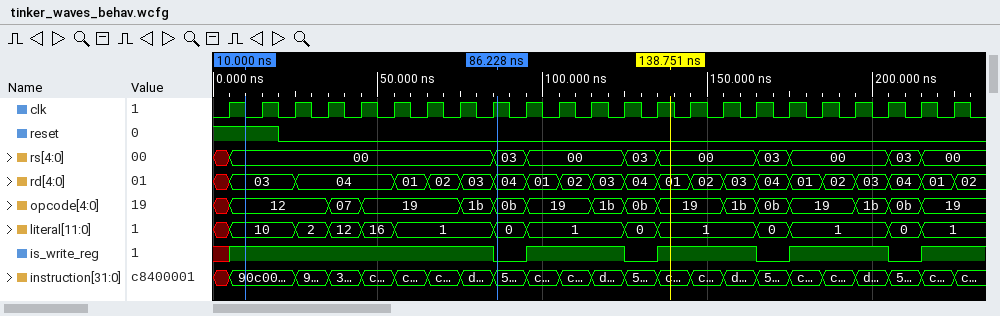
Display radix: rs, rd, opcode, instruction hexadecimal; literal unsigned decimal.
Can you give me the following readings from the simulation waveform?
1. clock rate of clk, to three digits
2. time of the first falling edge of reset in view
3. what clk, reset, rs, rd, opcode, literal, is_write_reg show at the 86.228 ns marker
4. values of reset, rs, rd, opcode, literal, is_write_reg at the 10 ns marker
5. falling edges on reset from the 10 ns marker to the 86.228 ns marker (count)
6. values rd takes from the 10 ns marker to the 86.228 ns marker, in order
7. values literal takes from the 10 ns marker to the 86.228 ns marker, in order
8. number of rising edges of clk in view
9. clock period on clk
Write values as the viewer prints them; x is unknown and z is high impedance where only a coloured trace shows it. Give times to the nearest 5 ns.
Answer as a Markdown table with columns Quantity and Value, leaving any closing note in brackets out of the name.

| Quantity | Value |
|---|---|
| clock rate of clk, to three digits | 100 MHz |
| time of the first falling edge of reset in view | 20 ns |
| what clk, reset, rs, rd, opcode, literal, is_write_reg show at the 86.228 ns marker | clk=1, reset=0, rs=03, rd=04, opcode=0b, literal=0, is_write_reg=0 |
| values of reset, rs, rd, opcode, literal, is_write_reg at the 10 ns marker | reset=1, rs=00, rd=03, opcode=12, literal=10, is_write_reg=1 |
| falling edges on reset from the 10 ns marker to the 86.228 ns marker | 1 |
| values rd takes from the 10 ns marker to the 86.228 ns marker, in order | 03, 04, 01, 02, 03, 04 |
| values literal takes from the 10 ns marker to the 86.228 ns marker, in order | 10, 2, 12, 16, 1, 0 |
| number of rising edges of clk in view | 23 |
| clock period on clk | 10 ns |
